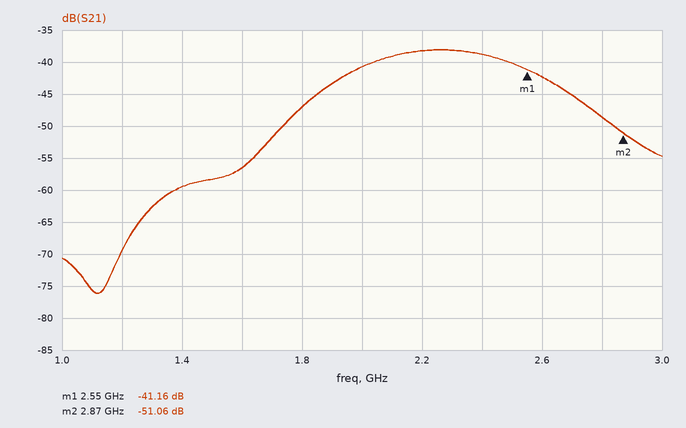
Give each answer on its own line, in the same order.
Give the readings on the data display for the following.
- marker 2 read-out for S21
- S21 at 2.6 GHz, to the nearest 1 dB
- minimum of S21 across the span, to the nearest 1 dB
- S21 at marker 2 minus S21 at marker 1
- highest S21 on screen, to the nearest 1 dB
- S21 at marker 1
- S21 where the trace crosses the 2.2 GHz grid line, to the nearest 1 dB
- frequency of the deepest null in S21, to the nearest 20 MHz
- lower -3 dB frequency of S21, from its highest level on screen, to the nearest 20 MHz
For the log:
-51.06 dB
-42 dB
-76 dB
-9.90 dB
-38 dB
-41.16 dB
-38 dB
1.12 GHz
1.98 GHz
